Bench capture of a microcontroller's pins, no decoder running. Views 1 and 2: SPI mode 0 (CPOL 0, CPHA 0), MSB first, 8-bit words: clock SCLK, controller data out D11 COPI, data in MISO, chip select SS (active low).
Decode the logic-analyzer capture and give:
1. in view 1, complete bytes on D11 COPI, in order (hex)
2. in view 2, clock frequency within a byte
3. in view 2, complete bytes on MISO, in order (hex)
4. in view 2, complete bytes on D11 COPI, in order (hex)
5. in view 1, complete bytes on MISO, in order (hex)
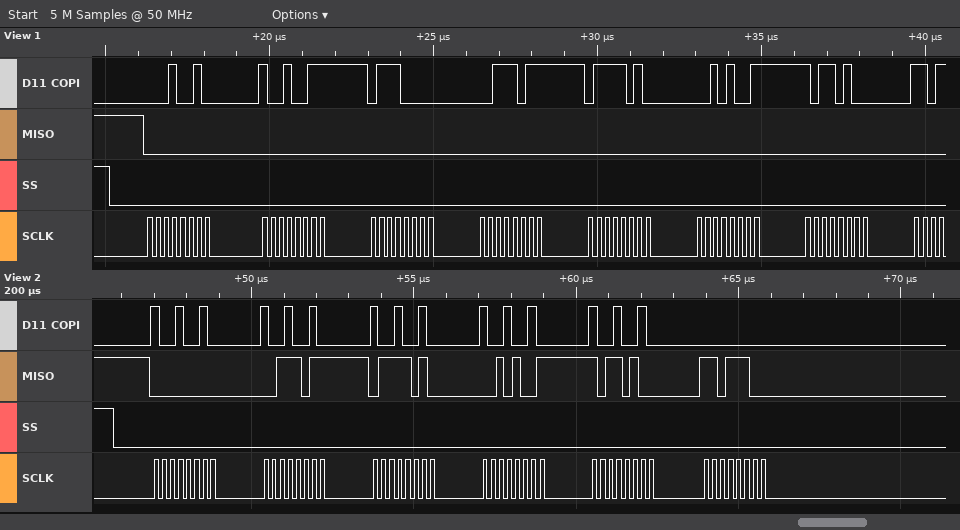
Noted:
12 93 70 3B 7A 29 B4
4 MHz
00 3B 7A 29 B4 DC
92 92 92 92 92 00
00 00 00 00 00 00 00
